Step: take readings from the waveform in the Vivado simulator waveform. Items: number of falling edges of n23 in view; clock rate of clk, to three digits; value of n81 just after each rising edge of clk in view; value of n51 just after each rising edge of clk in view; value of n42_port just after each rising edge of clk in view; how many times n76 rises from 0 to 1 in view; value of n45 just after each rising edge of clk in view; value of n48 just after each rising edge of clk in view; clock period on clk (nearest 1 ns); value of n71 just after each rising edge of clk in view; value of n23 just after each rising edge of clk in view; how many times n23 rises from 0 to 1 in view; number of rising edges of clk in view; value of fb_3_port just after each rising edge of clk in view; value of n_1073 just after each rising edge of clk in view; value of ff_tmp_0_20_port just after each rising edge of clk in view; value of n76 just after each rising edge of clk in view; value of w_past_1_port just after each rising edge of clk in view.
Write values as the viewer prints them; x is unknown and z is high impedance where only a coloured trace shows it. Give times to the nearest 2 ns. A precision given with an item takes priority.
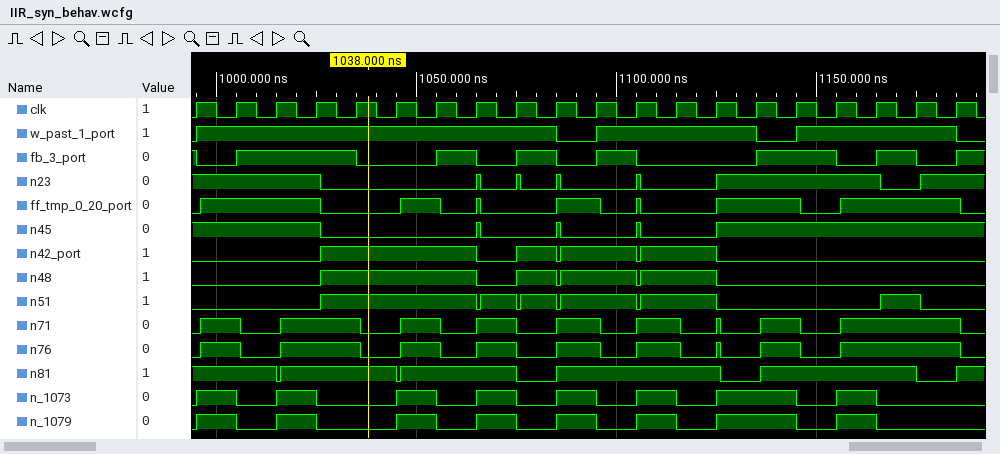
6
100 MHz
1 1 0 1 1 0 1 1 0 1 1 1 1 1 0 1 1 1 0 1
0 0 0 0 1 1 1 0 0 0 1 0 1 0 0 0 0 0 1 0
0 0 0 0 1 1 1 0 1 0 1 0 1 0 0 0 0 0 0 0
9
1 1 1 1 0 0 0 1 0 1 0 1 0 1 1 1 1 1 1 1
0 0 0 0 1 1 1 0 1 0 1 0 1 0 0 0 0 0 0 0
10 ns
0 1 0 1 1 0 1 1 0 1 1 1 1 1 0 1 0 1 1 1
1 1 1 1 0 0 0 1 1 1 0 1 0 1 1 1 1 1 0 1
6
20
0 1 1 1 0 0 1 0 1 0 1 0 0 0 1 1 0 1 0 1
1 0 1 0 0 1 0 1 0 1 0 1 0 1 1 0 1 0 0 0
0 1 1 1 0 0 1 1 0 1 1 1 0 1 1 1 0 1 1 1
0 1 0 1 1 0 1 1 0 1 1 1 1 1 0 1 0 1 1 1
1 1 1 1 1 1 1 1 1 0 1 1 1 1 0 1 1 1 1 0
